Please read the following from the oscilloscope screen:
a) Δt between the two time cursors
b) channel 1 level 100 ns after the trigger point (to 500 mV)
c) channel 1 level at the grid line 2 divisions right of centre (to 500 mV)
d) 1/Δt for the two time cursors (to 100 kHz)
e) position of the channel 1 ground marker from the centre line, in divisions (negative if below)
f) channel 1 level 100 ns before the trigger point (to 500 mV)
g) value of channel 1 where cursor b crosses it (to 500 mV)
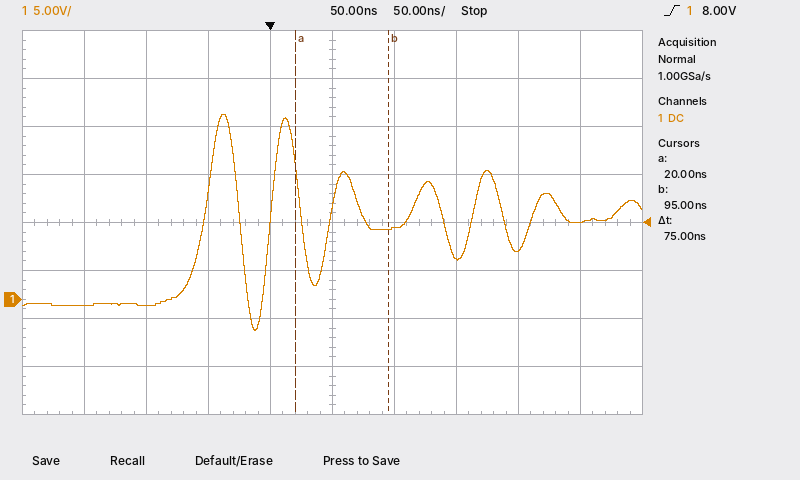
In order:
75 ns
7.5 V
4.5 V
13.3 MHz
-1.6 div
-500 mV
7.5 V
